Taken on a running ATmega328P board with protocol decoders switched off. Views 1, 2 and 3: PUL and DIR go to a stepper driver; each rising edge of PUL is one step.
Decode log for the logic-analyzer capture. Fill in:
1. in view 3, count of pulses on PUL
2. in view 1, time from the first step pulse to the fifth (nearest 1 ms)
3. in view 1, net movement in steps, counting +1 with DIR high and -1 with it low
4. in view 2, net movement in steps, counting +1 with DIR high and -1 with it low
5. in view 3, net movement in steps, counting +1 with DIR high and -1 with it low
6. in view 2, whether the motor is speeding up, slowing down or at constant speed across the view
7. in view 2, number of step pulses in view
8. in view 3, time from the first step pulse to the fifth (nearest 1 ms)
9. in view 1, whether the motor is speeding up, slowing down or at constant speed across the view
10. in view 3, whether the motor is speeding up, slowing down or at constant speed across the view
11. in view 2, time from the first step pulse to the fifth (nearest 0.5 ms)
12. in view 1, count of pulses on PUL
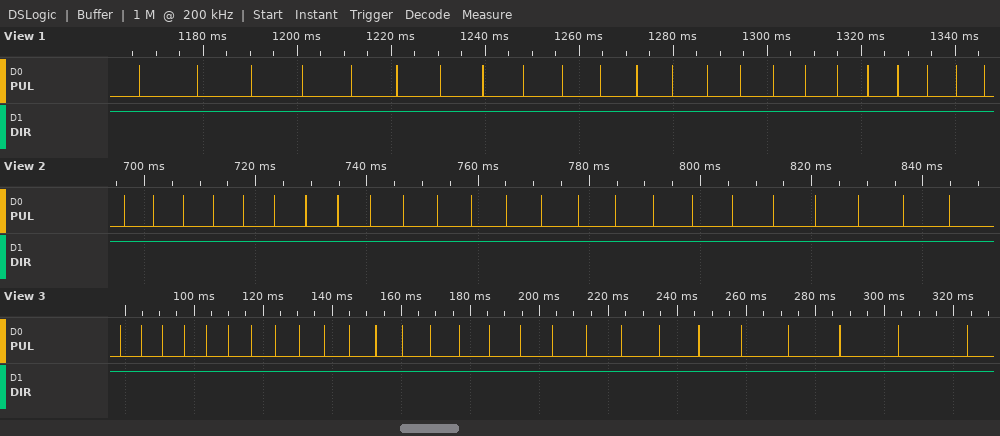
27
45 ms
+23
+24
+27
slowing down
24
25 ms
speeding up
slowing down
21.5 ms
23
